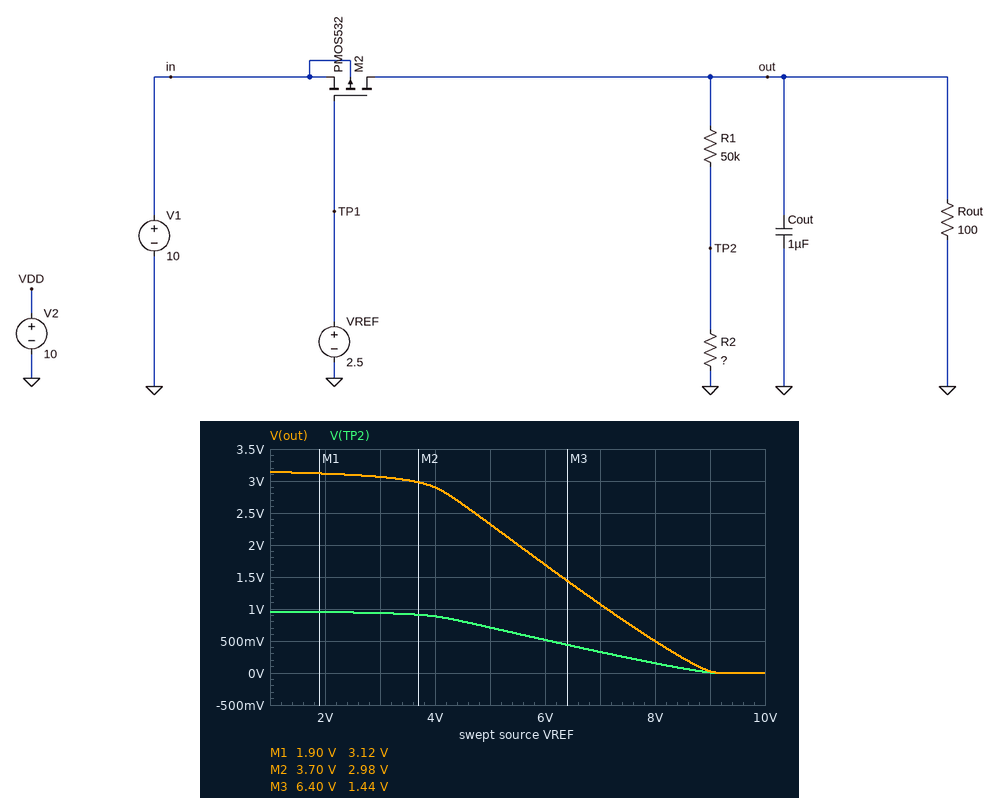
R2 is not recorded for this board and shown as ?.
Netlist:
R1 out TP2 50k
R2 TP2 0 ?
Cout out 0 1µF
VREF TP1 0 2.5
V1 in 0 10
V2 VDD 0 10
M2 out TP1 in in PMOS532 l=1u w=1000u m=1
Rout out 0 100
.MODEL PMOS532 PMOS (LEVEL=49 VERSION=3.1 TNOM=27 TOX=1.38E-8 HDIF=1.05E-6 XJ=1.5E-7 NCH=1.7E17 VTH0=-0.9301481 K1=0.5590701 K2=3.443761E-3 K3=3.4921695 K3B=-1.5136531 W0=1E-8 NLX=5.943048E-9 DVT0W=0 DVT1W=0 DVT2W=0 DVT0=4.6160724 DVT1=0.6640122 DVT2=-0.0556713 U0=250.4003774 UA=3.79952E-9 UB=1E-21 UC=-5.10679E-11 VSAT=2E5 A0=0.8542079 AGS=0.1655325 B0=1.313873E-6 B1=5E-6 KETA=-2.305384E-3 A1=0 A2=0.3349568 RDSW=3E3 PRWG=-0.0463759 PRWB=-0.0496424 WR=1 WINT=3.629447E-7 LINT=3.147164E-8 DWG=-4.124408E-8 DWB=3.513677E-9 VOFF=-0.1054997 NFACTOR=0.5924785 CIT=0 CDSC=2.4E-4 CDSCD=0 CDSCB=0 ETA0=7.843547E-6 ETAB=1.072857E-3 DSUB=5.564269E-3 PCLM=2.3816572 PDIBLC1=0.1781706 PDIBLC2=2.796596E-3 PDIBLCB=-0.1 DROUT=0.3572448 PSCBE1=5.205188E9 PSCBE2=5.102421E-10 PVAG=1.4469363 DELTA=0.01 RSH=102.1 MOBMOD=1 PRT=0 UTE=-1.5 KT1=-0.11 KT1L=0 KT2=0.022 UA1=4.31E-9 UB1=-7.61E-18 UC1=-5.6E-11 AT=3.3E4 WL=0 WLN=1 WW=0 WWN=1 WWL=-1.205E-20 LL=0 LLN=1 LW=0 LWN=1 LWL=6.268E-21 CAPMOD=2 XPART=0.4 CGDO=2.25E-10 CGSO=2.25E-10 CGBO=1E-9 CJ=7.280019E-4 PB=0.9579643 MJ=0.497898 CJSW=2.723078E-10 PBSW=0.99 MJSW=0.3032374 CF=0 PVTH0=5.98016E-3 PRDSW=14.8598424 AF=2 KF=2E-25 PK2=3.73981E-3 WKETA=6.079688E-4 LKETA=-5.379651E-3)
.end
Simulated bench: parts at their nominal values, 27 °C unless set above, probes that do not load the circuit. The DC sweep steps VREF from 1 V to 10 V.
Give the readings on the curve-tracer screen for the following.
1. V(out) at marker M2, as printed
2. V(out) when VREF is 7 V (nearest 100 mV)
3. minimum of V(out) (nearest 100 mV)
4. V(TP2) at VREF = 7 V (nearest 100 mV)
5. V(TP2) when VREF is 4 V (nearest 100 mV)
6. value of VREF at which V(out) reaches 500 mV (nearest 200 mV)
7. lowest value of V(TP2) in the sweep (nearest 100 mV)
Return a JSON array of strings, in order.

["2.98 V", "1.1 V", "0 V", "300 mV", "900 mV", "8.0 V", "0 V"]
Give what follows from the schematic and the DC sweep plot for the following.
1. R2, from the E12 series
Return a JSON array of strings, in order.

["22 kΩ"]
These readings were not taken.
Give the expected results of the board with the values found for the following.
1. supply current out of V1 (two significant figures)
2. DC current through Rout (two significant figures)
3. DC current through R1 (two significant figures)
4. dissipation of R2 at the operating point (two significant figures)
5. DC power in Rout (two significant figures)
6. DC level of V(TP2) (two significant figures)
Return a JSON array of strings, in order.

["31 mA", "31 mA", "43 µA", "41 µW", "96 mW", "950 mV"]
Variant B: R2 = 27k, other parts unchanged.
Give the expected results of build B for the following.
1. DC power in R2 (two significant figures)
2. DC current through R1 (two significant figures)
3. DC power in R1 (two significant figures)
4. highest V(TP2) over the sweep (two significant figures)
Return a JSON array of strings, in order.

["44 µW", "40 µA", "81 µW", "1.1 V"]
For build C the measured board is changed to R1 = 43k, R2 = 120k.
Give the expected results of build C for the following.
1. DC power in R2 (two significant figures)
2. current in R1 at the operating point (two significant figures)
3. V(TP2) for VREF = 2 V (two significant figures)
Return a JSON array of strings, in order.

["43 µW", "19 µA", "2.3 V"]
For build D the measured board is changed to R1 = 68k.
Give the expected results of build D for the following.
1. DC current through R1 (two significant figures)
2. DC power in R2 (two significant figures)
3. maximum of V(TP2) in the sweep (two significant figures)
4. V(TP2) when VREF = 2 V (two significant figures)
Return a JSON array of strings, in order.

["34 µA", "26 µW", "770 mV", "760 mV"]
